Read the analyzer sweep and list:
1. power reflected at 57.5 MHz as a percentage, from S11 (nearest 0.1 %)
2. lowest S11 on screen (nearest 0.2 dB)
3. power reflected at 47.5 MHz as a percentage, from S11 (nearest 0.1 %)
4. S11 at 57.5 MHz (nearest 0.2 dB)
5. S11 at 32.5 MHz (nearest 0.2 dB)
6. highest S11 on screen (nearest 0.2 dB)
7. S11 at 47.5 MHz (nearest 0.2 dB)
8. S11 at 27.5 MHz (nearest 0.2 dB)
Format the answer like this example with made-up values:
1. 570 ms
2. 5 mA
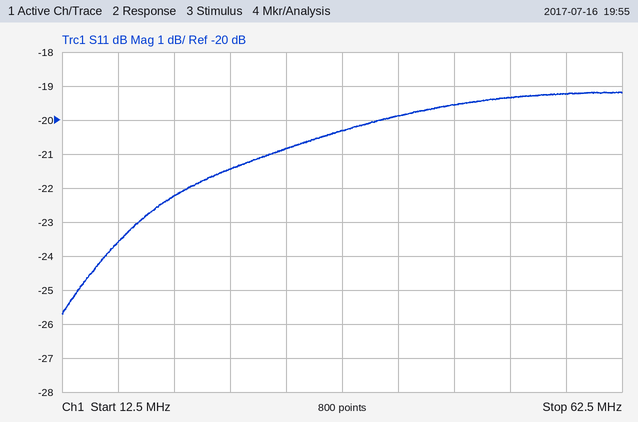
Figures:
1. 1.2 %
2. -25.8 dB
3. 1.1 %
4. -19.2 dB
5. -20.8 dB
6. -19.2 dB
7. -19.6 dB
8. -21.4 dB
